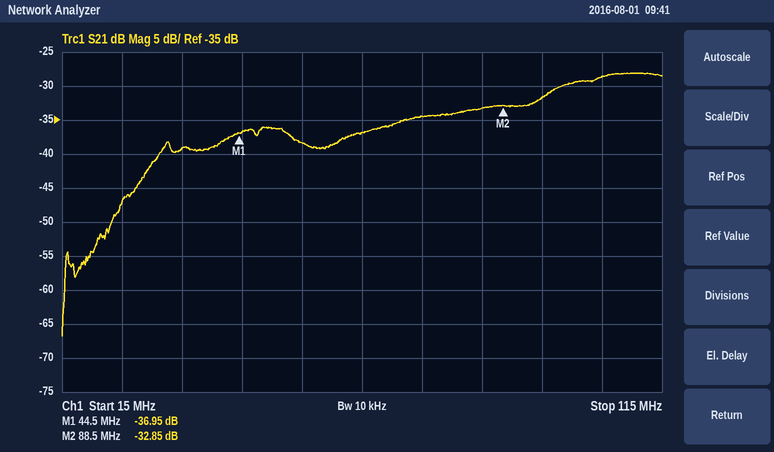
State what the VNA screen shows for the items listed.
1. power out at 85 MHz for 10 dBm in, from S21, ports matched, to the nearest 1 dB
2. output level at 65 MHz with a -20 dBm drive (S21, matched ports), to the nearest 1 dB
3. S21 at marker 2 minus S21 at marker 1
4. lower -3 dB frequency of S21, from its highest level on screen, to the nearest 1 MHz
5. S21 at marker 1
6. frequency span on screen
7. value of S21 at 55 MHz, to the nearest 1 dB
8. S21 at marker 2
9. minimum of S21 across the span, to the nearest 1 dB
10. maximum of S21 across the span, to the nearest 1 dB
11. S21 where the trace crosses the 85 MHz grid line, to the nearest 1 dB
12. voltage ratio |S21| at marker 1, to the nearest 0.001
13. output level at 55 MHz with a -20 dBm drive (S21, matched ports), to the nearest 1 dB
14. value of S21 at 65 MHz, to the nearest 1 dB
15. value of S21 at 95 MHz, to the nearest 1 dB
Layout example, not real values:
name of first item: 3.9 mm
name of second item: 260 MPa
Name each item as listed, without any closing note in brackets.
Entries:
power out at 85 MHz for 10 dBm in, from S21, ports matched, to the nearest 1 dB: -23 dBm
output level at 65 MHz with a -20 dBm drive (S21, matched ports), to the nearest 1 dB: -57 dBm
S21 at marker 2 minus S21 at marker 1: 4.10 dB
lower -3 dB frequency of S21, from its highest level on screen, to the nearest 1 MHz: 96 MHz
S21 at marker 1: -36.95 dB
frequency span on screen: 100 MHz
value of S21 at 55 MHz, to the nearest 1 dB: -38 dB
S21 at marker 2: -32.85 dB
minimum of S21 across the span, to the nearest 1 dB: -67 dB
maximum of S21 across the span, to the nearest 1 dB: -28 dB
S21 where the trace crosses the 85 MHz grid line, to the nearest 1 dB: -33 dB
voltage ratio |S21| at marker 1, to the nearest 0.001: 0.014
output level at 55 MHz with a -20 dBm drive (S21, matched ports), to the nearest 1 dB: -58 dBm
value of S21 at 65 MHz, to the nearest 1 dB: -37 dB
value of S21 at 95 MHz, to the nearest 1 dB: -32 dB
